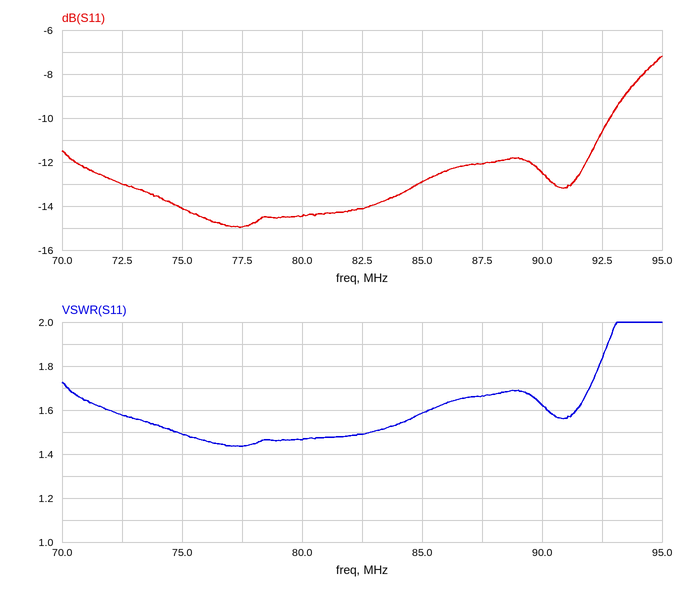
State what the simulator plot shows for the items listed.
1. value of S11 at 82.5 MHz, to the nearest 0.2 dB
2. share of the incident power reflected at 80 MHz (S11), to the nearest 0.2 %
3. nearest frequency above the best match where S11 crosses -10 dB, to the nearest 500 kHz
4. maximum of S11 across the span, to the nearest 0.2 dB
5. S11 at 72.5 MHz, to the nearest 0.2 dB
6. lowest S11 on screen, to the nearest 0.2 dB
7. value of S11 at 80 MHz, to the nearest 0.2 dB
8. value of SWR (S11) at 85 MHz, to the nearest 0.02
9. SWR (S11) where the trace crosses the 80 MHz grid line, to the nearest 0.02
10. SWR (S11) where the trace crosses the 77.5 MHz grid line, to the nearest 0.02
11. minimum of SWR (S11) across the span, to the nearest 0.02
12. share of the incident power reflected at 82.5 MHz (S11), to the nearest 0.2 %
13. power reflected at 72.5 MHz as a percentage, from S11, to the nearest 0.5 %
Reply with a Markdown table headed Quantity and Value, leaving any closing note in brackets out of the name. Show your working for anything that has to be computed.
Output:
| Quantity | Value |
|---|---|
| value of S11 at 82.5 MHz, to the nearest 0.2 dB | -14.2 dB |
| share of the incident power reflected at 80 MHz (S11), to the nearest 0.2 % | 10^(-14.4/10) ≈ 3.6 % |
| nearest frequency above the best match where S11 crosses -10 dB, to the nearest 500 kHz | 93.0 MHz |
| maximum of S11 across the span, to the nearest 0.2 dB | -7.2 dB |
| S11 at 72.5 MHz, to the nearest 0.2 dB | -13.0 dB |
| lowest S11 on screen, to the nearest 0.2 dB | -15.0 dB |
| value of S11 at 80 MHz, to the nearest 0.2 dB | -14.4 dB |
| value of SWR (S11) at 85 MHz, to the nearest 0.02 | 1.58 |
| SWR (S11) where the trace crosses the 80 MHz grid line, to the nearest 0.02 | 1.46 |
| SWR (S11) where the trace crosses the 77.5 MHz grid line, to the nearest 0.02 | 1.44 |
| minimum of SWR (S11) across the span, to the nearest 0.02 | 1.44 |
| share of the incident power reflected at 82.5 MHz (S11), to the nearest 0.2 % | 10^(-14.2/10) ≈ 3.8 % |
| power reflected at 72.5 MHz as a percentage, from S11, to the nearest 0.5 % | 10^(-13/10) ≈ 5.0 % |
